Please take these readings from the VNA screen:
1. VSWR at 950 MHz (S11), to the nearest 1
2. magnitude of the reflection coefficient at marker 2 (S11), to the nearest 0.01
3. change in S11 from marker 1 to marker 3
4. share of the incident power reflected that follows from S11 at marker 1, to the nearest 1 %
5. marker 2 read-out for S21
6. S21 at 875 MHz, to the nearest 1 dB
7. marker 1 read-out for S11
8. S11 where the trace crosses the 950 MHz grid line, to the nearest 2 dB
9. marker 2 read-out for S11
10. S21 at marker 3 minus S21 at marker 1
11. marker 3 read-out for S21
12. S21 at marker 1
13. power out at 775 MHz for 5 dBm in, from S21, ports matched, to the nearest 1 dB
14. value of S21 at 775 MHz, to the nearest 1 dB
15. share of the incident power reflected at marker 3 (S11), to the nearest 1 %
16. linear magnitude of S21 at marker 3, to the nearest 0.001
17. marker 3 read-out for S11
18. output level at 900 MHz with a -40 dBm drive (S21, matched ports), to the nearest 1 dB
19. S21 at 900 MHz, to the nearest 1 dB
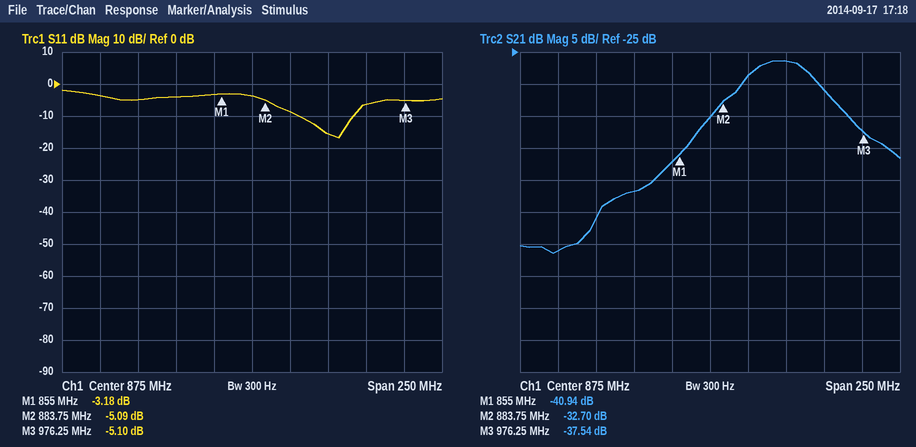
3
0.56
-1.92 dB
48 %
-32.70 dB
-35 dB
-3.18 dB
-6 dB
-5.09 dB
3.40 dB
-37.54 dB
-40.94 dB
-51 dBm
-56 dB
31 %
0.013
-5.10 dB
-69 dBm
-29 dB
